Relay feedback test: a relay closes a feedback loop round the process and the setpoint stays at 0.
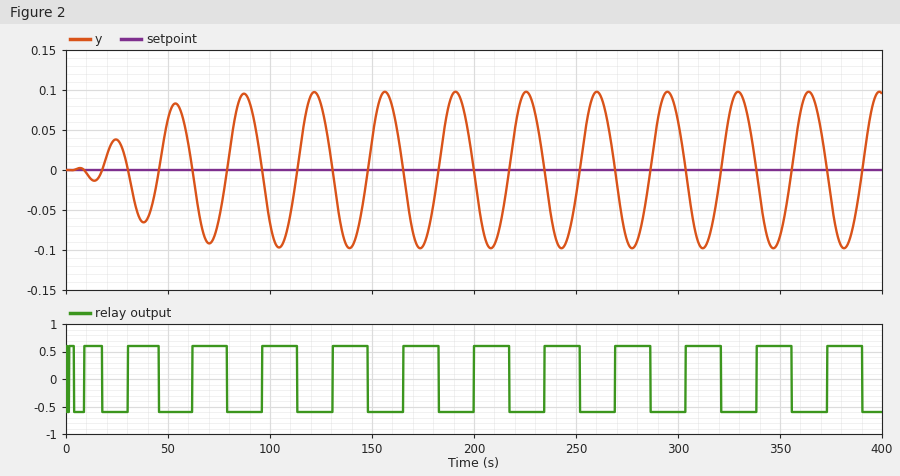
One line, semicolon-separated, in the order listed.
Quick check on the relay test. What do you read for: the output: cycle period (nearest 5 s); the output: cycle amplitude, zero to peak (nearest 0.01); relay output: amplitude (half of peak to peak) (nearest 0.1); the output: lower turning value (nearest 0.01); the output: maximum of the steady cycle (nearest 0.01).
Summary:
35 s; 0.10; 0.6; -0.10; 0.10
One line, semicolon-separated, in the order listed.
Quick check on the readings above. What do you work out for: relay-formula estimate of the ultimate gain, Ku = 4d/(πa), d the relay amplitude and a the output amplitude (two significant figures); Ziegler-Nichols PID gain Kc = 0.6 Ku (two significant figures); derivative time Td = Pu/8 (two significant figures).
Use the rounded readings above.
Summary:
7.6; 4.6; 4.4 s
